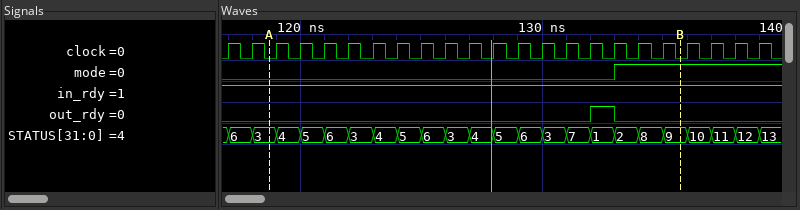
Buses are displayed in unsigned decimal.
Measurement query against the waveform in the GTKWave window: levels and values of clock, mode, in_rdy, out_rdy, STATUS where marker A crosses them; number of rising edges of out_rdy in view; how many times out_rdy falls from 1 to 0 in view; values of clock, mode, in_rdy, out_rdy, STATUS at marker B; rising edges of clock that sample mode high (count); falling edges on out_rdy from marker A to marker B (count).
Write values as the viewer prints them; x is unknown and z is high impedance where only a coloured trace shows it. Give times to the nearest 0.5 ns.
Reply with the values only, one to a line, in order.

clock=0, mode=0, in_rdy=1, out_rdy=0, STATUS=3
1
1
clock=0, mode=1, in_rdy=1, out_rdy=0, STATUS=9
6
1
